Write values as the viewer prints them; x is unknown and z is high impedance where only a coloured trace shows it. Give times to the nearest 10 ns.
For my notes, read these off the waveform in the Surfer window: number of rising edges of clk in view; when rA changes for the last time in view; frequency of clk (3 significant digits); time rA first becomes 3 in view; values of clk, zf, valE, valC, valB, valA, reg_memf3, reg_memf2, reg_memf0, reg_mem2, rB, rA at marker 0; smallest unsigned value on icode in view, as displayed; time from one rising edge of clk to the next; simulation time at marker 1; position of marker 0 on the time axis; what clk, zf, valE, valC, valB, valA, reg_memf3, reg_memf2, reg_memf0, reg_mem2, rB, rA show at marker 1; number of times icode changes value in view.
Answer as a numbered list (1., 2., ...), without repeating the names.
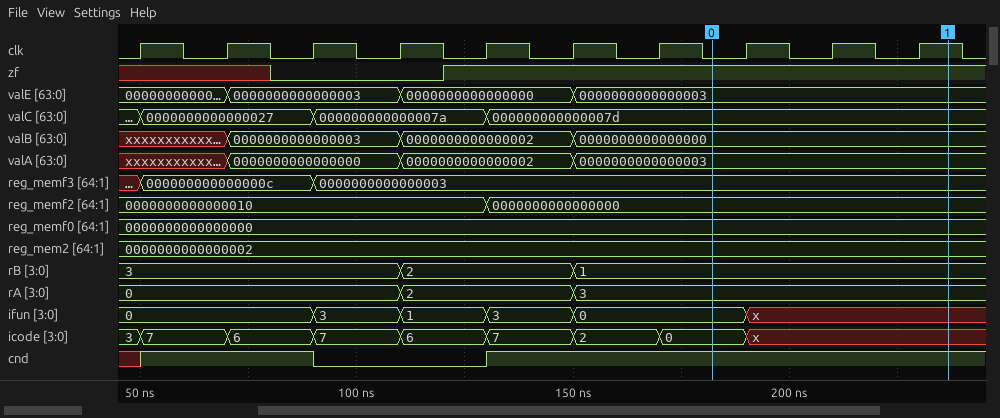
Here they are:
1. 10
2. 150 ns
3. 50.0 MHz
4. 150 ns
5. clk=0, zf=1, valE=0000000000000003, valC=000000000000007d, valB=0000000000000000, valA=0000000000000003, reg_memf3=0000000000000003, reg_memf2=0000000000000000, reg_memf0=0000000000000000, reg_mem2=0000000000000002, rB=1, rA=3
6. 0
7. 20 ns
8. 240 ns
9. 180 ns
10. clk=1, zf=1, valE=0000000000000003, valC=000000000000007d, valB=0000000000000000, valA=0000000000000003, reg_memf3=0000000000000003, reg_memf2=0000000000000000, reg_memf0=0000000000000000, reg_mem2=0000000000000002, rB=1, rA=3
11. 8
